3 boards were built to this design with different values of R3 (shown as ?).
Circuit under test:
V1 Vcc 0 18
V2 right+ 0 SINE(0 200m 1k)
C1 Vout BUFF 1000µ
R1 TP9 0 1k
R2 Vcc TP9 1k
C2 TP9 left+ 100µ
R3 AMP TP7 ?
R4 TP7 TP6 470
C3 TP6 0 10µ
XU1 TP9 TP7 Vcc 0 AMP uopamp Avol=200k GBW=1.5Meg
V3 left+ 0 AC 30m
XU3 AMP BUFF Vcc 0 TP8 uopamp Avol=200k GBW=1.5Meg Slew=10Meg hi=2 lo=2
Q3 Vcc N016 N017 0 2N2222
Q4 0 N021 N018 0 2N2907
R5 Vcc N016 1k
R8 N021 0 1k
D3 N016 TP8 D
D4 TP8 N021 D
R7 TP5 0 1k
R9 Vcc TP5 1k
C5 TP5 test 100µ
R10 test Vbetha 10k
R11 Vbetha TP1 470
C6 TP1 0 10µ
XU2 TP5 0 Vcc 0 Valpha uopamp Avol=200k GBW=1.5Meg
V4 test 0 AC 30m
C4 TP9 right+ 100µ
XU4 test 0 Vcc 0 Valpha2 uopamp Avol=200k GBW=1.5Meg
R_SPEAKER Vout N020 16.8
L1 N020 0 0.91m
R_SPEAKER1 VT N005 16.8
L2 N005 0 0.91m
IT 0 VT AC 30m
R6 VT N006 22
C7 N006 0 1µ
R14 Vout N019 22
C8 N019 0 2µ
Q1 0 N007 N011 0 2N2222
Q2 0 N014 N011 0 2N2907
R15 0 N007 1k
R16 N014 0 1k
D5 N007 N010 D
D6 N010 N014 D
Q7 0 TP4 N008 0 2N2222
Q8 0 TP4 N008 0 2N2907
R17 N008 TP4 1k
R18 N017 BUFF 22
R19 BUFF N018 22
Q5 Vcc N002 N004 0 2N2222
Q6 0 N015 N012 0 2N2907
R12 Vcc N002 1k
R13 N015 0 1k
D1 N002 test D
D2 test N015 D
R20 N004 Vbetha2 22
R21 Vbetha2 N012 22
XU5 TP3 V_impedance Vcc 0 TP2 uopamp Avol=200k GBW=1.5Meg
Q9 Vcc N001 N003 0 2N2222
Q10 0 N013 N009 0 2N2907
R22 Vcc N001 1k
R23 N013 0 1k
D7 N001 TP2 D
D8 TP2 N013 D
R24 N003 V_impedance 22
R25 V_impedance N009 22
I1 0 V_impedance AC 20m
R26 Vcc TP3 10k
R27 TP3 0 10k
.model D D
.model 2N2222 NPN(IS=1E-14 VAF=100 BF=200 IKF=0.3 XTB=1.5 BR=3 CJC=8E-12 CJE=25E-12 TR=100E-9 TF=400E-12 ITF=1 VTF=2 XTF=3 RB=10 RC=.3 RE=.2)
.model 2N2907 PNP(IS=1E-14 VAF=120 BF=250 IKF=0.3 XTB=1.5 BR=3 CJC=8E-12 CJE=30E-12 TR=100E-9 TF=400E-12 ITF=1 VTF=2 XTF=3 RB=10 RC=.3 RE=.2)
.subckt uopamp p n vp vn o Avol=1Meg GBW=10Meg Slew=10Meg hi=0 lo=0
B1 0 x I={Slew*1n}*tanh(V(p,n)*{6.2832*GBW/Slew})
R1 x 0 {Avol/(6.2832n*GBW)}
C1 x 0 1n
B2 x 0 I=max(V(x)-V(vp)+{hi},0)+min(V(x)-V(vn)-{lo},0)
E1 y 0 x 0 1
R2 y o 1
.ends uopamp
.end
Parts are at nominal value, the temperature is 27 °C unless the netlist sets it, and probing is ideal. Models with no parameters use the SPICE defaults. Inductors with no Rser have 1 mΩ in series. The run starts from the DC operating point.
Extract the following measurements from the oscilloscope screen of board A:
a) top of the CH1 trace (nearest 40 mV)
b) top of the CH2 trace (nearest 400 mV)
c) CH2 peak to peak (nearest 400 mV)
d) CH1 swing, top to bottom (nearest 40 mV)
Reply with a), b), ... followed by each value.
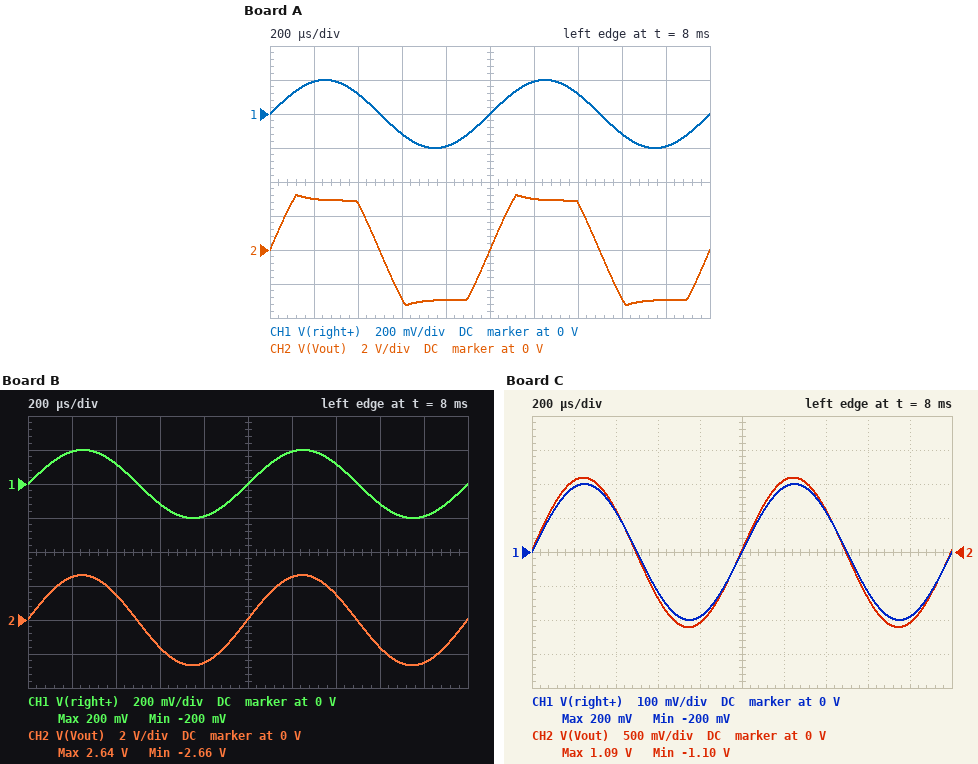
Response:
a) 200 mV
b) 3.2 V
c) 6.4 V
d) 400 mV
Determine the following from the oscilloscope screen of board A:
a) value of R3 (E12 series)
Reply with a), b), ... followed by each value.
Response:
a) 22 kΩ
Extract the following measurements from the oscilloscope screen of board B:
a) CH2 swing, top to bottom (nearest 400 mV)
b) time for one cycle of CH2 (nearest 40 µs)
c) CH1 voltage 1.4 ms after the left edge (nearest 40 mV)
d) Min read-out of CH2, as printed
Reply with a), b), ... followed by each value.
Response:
a) 5.2 V
b) 1.00 ms
c) 120 mV
d) -2.66 V
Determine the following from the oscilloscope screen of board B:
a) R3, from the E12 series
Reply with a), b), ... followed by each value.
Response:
a) 12 kΩ
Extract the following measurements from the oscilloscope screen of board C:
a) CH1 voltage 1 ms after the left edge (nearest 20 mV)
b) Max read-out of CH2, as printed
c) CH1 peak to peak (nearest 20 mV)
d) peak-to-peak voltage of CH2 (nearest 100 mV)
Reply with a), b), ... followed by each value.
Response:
a) 0 V
b) 1.09 V
c) 400 mV
d) 2.2 V
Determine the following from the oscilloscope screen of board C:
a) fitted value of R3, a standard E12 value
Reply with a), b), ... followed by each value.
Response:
a) 4.7 kΩ
